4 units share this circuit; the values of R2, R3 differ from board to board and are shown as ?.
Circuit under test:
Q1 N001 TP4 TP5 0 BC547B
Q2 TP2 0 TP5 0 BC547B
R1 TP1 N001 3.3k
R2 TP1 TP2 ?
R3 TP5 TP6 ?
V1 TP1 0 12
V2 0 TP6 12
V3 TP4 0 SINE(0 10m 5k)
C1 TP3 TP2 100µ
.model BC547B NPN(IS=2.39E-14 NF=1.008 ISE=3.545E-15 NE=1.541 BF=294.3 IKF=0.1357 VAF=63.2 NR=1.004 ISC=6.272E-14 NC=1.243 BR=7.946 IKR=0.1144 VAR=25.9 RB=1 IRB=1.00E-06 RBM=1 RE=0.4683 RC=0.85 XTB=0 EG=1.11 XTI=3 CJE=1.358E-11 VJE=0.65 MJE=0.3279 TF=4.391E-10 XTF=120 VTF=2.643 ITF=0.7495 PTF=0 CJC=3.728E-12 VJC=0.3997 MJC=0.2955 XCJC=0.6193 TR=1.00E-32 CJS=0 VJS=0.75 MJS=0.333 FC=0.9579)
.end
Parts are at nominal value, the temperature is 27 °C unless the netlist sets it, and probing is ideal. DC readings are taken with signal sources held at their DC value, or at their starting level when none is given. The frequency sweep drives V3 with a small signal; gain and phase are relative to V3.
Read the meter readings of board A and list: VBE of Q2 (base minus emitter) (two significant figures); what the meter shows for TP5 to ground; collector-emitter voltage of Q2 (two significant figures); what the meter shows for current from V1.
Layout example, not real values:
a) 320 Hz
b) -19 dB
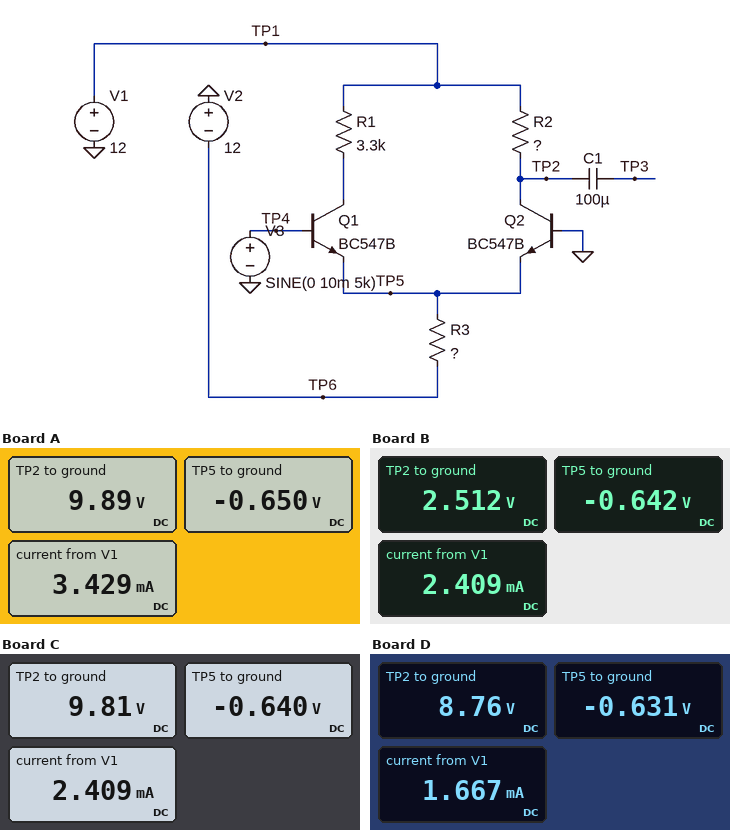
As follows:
a) 650 mV
b) -0.650 V
c) 11 V
d) 3.429 mA
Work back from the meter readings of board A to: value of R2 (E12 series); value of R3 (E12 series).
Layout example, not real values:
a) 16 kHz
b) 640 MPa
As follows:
a) 1.2 kΩ
b) 3.3 kΩ
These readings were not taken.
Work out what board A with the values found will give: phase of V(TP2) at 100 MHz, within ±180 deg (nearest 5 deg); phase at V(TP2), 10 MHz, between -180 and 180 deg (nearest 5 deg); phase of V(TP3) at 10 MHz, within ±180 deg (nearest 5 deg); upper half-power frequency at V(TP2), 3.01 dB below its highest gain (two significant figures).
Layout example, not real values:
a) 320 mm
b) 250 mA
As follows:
a) -50 deg
b) -5 deg
c) -5 deg
d) 96 MHz
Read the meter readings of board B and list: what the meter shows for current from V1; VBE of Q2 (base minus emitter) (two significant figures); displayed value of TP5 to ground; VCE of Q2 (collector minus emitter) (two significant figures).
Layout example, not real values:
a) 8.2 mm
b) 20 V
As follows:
a) 2.409 mA
b) 640 mV
c) -0.642 V
d) 3.2 V
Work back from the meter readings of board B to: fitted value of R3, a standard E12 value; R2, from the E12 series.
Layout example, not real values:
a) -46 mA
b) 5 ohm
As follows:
a) 4.7 kΩ
b) 8.2 kΩ
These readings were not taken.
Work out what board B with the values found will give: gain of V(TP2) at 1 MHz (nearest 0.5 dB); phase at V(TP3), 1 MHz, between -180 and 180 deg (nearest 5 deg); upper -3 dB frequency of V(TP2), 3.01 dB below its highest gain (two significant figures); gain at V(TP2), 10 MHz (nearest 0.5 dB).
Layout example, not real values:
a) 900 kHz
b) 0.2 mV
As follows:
a) 44.5 dB
b) -5 deg
c) 9.9 MHz
d) 41.5 dB
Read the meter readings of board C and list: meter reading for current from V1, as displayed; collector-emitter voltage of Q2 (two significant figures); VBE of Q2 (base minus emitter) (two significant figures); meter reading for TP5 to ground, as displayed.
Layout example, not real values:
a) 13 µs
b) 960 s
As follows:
a) 2.409 mA
b) 10 V
c) 640 mV
d) -0.640 V
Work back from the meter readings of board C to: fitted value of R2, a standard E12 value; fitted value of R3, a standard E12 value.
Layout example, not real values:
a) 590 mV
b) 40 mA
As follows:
a) 1.8 kΩ
b) 4.7 kΩ
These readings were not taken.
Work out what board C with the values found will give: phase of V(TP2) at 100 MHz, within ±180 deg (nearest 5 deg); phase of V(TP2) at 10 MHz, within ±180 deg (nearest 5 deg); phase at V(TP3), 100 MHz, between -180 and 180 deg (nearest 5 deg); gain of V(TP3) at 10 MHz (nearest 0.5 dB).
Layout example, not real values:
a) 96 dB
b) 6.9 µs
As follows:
a) -60 deg
b) -10 deg
c) -60 deg
d) 31.5 dB
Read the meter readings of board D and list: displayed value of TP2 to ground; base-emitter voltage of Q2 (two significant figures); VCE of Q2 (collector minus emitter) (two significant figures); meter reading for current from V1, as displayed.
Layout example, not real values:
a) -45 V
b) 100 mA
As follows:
a) 8.76 V
b) 630 mV
c) 9.4 V
d) 1.667 mA
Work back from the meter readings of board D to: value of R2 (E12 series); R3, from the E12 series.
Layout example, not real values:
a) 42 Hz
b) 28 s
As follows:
a) 3.9 kΩ
b) 6.8 kΩ
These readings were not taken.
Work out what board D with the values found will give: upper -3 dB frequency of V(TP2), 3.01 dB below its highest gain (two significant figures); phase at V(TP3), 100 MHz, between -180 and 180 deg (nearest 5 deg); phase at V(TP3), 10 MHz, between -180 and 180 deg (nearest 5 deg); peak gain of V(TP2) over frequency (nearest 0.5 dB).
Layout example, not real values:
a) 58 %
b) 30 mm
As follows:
a) 28 MHz
b) -75 deg
c) -20 deg
d) 35.5 dB
